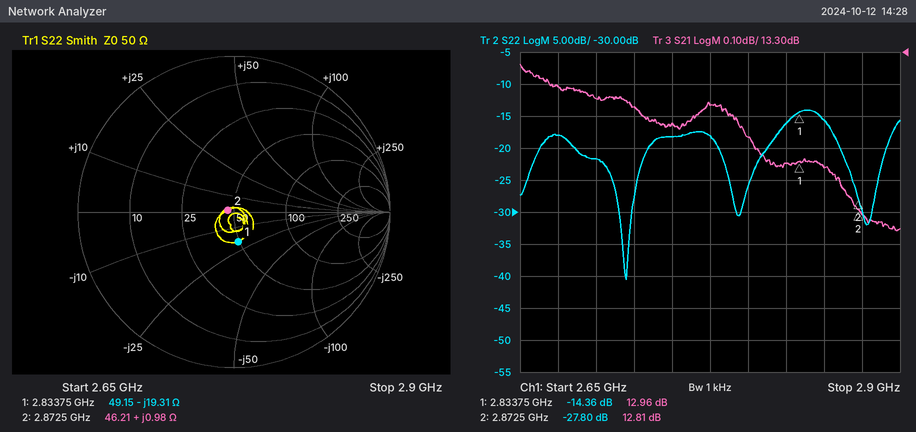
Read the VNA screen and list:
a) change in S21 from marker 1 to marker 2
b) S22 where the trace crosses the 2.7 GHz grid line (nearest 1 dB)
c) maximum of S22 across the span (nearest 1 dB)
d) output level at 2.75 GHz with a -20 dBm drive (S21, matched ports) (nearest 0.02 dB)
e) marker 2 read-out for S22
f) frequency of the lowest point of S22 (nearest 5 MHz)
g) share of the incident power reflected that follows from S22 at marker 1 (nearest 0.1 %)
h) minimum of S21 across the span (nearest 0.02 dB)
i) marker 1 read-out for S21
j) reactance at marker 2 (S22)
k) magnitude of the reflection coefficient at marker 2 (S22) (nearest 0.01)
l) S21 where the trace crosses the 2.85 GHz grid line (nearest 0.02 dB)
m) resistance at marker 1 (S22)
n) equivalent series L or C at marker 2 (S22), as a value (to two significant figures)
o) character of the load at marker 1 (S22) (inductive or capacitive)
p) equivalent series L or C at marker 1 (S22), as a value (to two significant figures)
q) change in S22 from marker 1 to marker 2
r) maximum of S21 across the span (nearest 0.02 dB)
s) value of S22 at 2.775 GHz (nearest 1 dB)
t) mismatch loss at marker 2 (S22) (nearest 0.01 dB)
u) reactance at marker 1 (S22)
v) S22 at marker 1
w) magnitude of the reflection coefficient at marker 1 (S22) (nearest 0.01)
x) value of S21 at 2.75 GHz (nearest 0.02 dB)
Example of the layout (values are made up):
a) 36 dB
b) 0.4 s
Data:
a) -0.15 dB
b) -22 dB
c) -14 dB
d) -6.92 dBm
e) -27.80 dB
f) 2.720 GHz
g) 3.7 %
h) 12.74 dB
i) 12.96 dB
j) +0.98 Ω
k) 0.04
l) 12.94 dB
m) 49.15 Ω
n) 54 pH
o) capacitive
p) 2.9 pF
q) -13.44 dB
r) 13.26 dB
s) -18 dB
t) 0.01 dB
u) -19.31 Ω
v) -14.36 dB
w) 0.19
x) 13.08 dB
